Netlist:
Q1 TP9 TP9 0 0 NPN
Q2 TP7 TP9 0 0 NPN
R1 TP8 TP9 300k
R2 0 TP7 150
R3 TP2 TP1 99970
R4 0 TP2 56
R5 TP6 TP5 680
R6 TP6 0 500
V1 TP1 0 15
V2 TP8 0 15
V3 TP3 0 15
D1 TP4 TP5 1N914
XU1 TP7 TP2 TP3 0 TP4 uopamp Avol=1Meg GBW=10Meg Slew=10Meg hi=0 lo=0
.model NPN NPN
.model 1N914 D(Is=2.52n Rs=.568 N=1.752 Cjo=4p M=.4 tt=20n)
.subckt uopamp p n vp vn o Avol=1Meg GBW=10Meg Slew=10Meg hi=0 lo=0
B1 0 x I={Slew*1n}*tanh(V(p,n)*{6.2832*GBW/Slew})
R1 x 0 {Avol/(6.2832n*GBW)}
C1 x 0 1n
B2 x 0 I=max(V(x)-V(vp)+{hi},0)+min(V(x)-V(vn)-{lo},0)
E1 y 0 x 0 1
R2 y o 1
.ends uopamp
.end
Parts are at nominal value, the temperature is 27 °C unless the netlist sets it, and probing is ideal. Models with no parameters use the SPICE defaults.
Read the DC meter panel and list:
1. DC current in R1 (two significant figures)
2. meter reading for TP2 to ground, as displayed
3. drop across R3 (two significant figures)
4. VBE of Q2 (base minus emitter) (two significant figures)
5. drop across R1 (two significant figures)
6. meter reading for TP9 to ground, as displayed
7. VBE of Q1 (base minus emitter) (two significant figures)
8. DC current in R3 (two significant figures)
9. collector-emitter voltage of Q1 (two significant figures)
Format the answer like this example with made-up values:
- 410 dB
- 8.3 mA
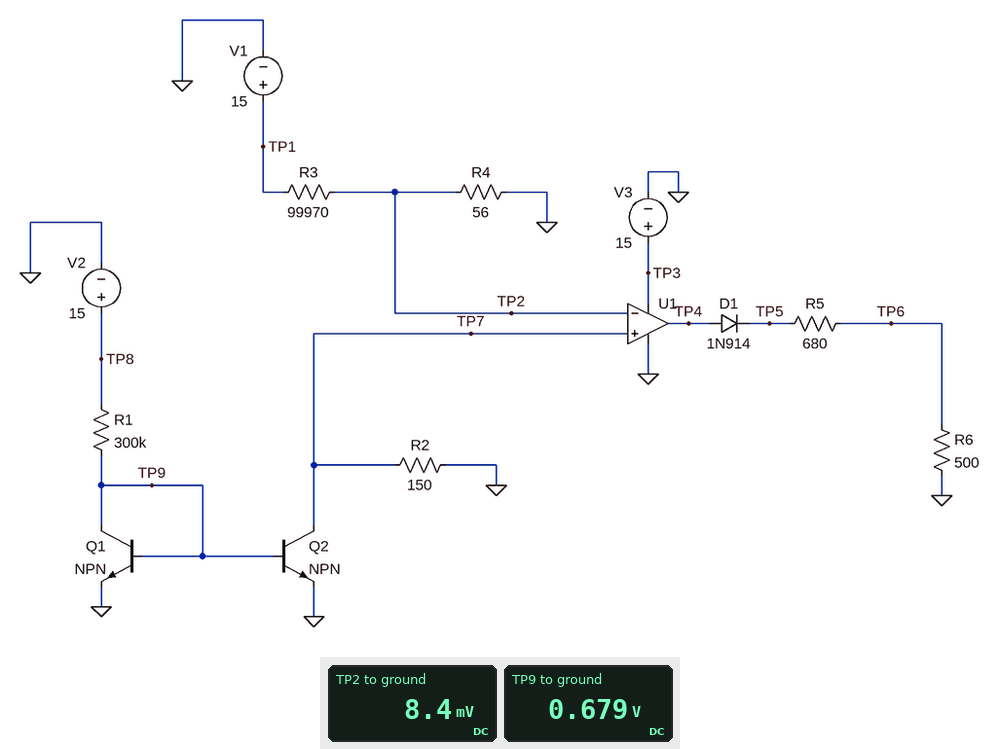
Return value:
- 48 µA
- 8.4 mV
- 15 V
- 680 mV
- 14 V
- 0.679 V
- 680 mV
- 150 µA
- 680 mV
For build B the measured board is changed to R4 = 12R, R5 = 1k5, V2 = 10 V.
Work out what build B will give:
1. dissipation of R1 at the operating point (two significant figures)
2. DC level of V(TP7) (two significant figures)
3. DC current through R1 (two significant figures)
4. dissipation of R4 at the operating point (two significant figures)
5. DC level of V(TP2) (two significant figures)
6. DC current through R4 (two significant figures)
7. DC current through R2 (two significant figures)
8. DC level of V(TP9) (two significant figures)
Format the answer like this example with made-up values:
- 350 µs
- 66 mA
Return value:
- 290 µW
- 2.0 mV
- 31 µA
- 270 nW
- 1.8 mV
- 150 µA
- 14 µA
- 670 mV
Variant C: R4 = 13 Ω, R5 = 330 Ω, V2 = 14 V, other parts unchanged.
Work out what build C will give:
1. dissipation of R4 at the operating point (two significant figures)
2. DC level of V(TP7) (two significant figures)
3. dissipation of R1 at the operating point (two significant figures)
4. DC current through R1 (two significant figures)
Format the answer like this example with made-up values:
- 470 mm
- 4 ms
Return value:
- 290 nW
- 2.8 mV
- 590 µW
- 44 µA
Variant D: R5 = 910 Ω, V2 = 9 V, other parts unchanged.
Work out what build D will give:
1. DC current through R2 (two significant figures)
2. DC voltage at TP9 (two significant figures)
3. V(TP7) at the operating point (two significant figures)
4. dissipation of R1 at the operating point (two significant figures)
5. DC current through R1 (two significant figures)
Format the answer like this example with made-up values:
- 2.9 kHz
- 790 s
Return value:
- 12 µA
- 660 mV
- 1.8 mV
- 230 µW
- 28 µA
